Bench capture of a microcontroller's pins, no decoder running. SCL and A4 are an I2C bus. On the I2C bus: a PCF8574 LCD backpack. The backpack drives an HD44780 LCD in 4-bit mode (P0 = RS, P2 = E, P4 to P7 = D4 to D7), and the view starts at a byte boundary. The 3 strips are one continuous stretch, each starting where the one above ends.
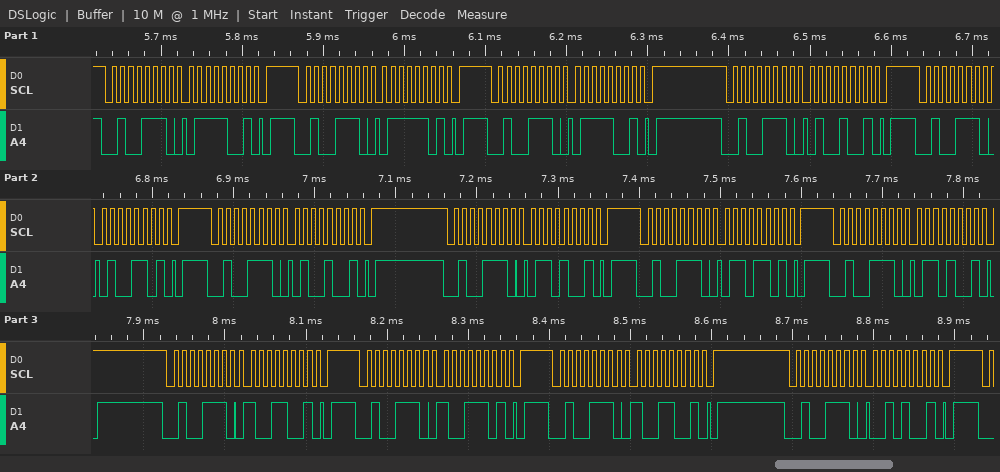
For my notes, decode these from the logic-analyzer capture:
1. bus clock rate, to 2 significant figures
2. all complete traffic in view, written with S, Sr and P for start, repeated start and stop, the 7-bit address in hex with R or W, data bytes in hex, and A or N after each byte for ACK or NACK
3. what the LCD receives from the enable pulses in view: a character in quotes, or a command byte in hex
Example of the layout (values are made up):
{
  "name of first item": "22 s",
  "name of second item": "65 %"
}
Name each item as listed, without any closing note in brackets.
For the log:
{
  "bus clock rate, to 2 significant figures": "100 kHz",
  "all complete traffic in view, written with S, Sr and P for start, repeated start and stop, the 7-bit address in hex with R or W, data bytes in hex, and A or N after each byte for ACK or NACK": "S 27W A 79 A P S 27W A 7D A P S 27W A 79 A P S 27W A 49 A P S 27W A 4D A P S 27W A 49 A P S 27W A 69 A P S 27W A 6D A P S 27W A 69 A P S 27W A 99 A P S 27W A 9D A P S 27W A 99 A P S 27W A 29 A P",
  "what the LCD receives from the enable pulses in view: a character in quotes, or a command byte in hex": "'t' 'i'"
}
